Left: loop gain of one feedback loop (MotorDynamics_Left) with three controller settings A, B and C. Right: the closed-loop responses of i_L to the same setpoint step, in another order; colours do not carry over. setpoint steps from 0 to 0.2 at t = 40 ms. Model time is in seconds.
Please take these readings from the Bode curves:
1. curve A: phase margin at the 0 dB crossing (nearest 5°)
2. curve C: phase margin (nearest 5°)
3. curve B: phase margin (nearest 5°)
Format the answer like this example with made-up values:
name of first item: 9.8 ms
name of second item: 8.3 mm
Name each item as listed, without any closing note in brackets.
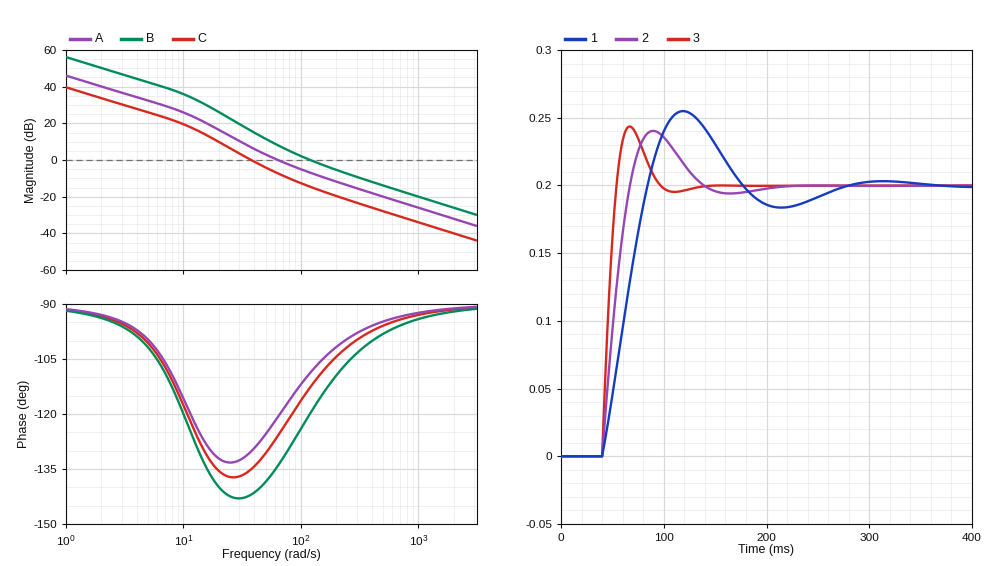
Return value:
curve A: phase margin at the 0 dB crossing: 60°
curve C: phase margin: 45°
curve B: phase margin: 60°
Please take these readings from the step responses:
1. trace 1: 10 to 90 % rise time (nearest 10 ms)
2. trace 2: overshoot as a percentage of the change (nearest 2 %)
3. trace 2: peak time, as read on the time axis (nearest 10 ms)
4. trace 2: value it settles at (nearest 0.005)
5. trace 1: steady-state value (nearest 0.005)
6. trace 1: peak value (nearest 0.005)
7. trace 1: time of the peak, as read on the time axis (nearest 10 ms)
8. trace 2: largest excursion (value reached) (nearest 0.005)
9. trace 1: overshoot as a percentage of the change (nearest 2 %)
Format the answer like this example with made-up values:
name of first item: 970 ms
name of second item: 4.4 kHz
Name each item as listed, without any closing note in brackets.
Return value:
trace 1: 10 to 90 % rise time: 30 ms
trace 2: overshoot as a percentage of the change: 20 %
trace 2: peak time, as read on the time axis: 90 ms
trace 2: value it settles at: 0.200
trace 1: steady-state value: 0.200
trace 1: peak value: 0.255
trace 1: time of the peak, as read on the time axis: 120 ms
trace 2: largest excursion (value reached): 0.240
trace 1: overshoot as a percentage of the change: 28 %
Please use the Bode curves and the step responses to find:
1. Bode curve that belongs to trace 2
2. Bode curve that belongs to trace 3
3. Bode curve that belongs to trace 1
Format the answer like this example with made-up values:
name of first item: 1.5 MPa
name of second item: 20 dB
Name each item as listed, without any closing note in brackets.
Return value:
Bode curve that belongs to trace 2: A
Bode curve that belongs to trace 3: B
Bode curve that belongs to trace 1: C
